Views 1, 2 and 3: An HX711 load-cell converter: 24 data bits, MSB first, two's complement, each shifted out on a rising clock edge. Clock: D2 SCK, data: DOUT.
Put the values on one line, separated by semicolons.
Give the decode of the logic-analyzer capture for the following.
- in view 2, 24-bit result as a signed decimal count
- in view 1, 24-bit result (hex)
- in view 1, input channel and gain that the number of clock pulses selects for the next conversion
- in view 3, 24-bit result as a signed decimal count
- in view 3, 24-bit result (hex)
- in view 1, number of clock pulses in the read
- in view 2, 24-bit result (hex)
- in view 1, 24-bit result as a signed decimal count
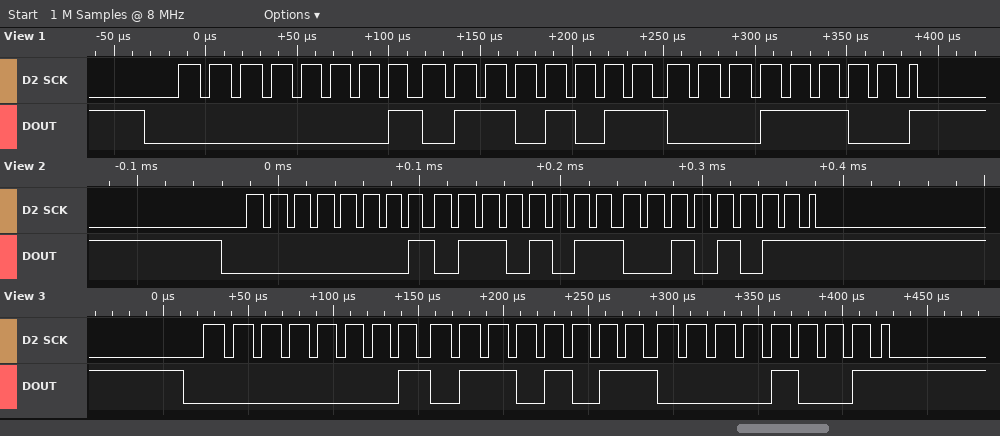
92971; 0x016B1C; channel A, gain 128; 92937; 0x016B09; 25; 0x016B2B; 92956
